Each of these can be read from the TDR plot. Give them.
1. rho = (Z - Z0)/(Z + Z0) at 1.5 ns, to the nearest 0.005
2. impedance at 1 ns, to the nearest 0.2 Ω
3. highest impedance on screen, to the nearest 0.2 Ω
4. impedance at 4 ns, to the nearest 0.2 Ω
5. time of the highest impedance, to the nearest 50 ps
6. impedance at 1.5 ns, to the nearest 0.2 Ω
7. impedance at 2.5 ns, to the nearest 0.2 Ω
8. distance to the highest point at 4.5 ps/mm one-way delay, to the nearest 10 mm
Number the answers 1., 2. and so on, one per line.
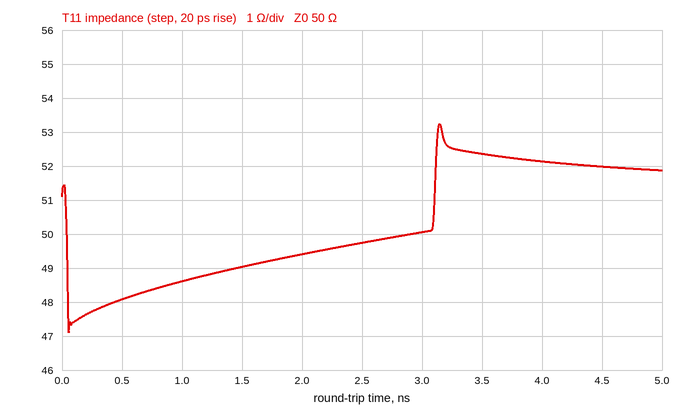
1. -0.010
2. 48.6 Ω
3. 53.2 Ω
4. 52.2 Ω
5. 3.15 ns
6. 49.0 Ω
7. 49.8 Ω
8. 350 mm
